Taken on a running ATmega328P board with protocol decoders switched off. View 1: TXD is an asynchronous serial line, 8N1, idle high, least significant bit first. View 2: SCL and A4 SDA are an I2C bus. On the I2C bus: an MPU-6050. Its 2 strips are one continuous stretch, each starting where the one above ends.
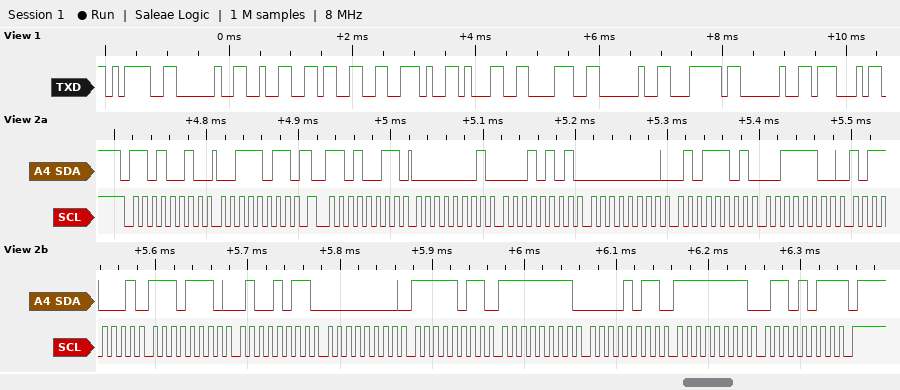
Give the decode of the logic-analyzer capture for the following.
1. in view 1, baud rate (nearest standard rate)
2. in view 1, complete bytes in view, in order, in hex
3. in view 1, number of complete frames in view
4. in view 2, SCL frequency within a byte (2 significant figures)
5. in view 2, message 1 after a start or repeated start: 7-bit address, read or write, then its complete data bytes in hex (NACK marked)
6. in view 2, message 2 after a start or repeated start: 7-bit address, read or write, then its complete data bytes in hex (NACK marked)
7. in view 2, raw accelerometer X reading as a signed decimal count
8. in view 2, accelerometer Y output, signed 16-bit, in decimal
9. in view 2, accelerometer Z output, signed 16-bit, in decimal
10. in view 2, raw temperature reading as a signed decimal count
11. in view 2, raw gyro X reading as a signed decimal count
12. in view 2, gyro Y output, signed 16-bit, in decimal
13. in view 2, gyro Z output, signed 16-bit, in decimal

9600 baud
3D 20 32 33 2E 31 38 20 7C 20 47
11
100 kHz
0x69 write: 3B
0x69 read: 01 15 00 5D 3C B1 EE 4B 00 FB FF 0B FF 6B NACK
277
93
15537
-4533
251
-245
-149
